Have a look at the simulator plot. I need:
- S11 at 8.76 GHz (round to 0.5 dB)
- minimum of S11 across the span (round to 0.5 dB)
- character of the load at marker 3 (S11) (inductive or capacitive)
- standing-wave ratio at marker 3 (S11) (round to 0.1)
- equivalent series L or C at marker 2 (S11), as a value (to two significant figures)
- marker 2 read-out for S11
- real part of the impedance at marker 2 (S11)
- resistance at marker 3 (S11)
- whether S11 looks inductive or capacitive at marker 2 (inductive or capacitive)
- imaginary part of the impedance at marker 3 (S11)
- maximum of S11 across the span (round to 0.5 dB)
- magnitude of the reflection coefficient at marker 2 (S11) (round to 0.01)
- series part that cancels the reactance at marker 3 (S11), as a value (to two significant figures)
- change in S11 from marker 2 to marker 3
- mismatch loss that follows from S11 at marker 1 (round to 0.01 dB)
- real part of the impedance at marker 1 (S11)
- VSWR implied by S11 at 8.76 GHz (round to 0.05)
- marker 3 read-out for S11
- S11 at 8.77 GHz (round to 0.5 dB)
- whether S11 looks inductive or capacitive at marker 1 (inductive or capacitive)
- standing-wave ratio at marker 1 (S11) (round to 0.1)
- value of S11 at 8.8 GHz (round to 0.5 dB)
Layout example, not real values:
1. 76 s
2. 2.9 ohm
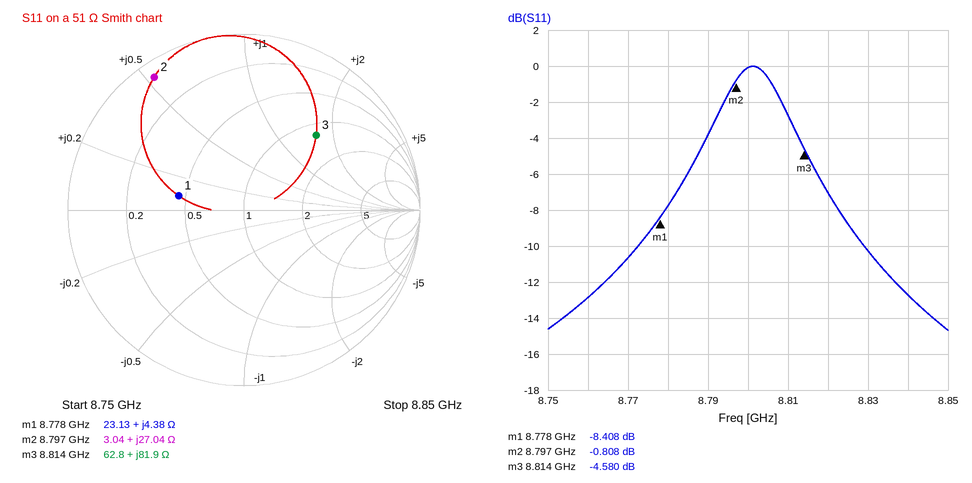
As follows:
1. -13.0 dB
2. -14.5 dB
3. inductive
4. 3.9
5. 490 pH
6. -0.808 dB
7. 3.04 Ω
8. 62.8 Ω
9. inductive
10. +81.9 Ω
11. 0.0 dB
12. 0.91
13. 220 fF
14. -3.772 dB
15. 0.68 dB
16. 23.13 Ω
17. 1.60
18. -4.580 dB
19. -10.5 dB
20. inductive
21. 2.2
22. 0.0 dB
